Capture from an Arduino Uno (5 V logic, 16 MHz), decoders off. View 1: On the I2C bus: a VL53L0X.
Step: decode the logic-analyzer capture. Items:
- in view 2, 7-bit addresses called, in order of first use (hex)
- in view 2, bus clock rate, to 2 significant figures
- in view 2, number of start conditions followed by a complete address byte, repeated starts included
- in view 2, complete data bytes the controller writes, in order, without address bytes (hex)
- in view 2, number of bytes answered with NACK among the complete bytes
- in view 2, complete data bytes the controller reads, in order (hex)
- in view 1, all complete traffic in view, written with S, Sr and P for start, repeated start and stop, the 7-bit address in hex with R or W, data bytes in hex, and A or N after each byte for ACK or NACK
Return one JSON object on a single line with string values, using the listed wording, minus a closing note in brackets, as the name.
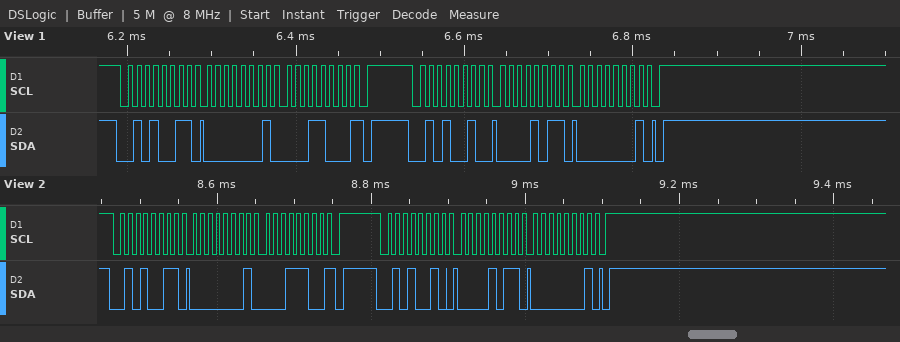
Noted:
{"in view 2, 7-bit addresses called, in order of first use": "0x29", "in view 2, bus clock rate, to 2 significant figures": "100 kHz", "in view 2, number of start conditions followed by a complete address byte, repeated starts included": "2", "in view 2, complete data bytes the controller writes, in order, without address bytes": "0B 01", "in view 2, number of bytes answered with NACK among the complete bytes": "1", "in view 2, complete data bytes the controller reads, in order": "01 1C", "in view 1, all complete traffic in view, written with S, Sr and P for start, repeated start and stop, the 7-bit address in hex with R or W, data bytes in hex, and A or N after each byte for ACK or NACK": "S 29R A 01 A 18 N P S 29W A 0B A 01 A P"}
